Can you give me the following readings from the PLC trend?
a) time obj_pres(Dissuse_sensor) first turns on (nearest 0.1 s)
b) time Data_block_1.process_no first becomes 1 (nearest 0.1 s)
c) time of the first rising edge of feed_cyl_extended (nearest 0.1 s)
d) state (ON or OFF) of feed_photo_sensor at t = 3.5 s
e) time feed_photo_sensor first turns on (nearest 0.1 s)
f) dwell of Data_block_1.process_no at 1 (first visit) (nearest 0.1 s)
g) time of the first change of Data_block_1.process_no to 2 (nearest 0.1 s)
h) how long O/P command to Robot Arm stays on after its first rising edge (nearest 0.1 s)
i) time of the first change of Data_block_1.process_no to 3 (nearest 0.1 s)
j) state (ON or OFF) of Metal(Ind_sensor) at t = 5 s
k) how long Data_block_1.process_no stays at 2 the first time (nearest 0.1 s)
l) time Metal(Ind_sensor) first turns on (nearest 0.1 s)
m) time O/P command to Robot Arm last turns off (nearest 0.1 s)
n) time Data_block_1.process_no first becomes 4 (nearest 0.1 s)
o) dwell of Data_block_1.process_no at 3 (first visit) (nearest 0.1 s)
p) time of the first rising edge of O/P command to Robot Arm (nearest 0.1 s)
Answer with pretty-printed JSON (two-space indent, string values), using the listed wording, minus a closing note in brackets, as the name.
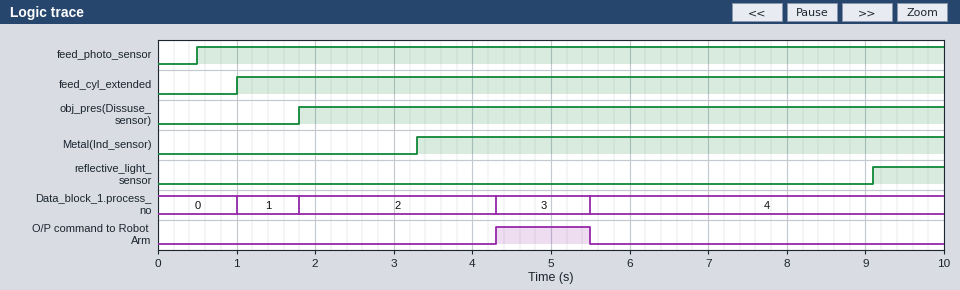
{
  "time obj_pres(Dissuse_sensor) first turns on": "1.8 s",
  "time Data_block_1.process_no first becomes 1": "1.0 s",
  "time of the first rising edge of feed_cyl_extended": "1.0 s",
  "state (ON or OFF) of feed_photo_sensor at t = 3.5 s": "ON",
  "time feed_photo_sensor first turns on": "0.5 s",
  "dwell of Data_block_1.process_no at 1 (first visit)": "0.8 s",
  "time of the first change of Data_block_1.process_no to 2": "1.8 s",
  "how long O/P command to Robot Arm stays on after its first rising edge": "1.2 s",
  "time of the first change of Data_block_1.process_no to 3": "4.3 s",
  "state (ON or OFF) of Metal(Ind_sensor) at t = 5 s": "ON",
  "how long Data_block_1.process_no stays at 2 the first time": "2.5 s",
  "time Metal(Ind_sensor) first turns on": "3.3 s",
  "time O/P command to Robot Arm last turns off": "5.5 s",
  "time Data_block_1.process_no first becomes 4": "5.5 s",
  "dwell of Data_block_1.process_no at 3 (first visit)": "1.2 s",
  "time of the first rising edge of O/P command to Robot Arm": "4.3 s"
}
